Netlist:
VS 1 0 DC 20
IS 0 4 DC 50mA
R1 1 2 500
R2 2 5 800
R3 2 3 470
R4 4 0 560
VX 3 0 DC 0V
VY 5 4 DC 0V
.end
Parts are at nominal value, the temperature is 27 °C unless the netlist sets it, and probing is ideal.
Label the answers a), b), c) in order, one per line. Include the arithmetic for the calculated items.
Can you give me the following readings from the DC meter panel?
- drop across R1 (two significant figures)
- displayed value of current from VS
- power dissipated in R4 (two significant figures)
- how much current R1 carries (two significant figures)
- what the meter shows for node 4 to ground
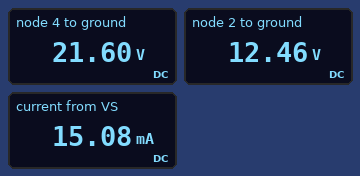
a) 20 V - 12.46 V = 7.5 V
b) 15.08 mA
c) (21.6 V)^2 / 560 Ω = 830 mW
d) (20 V - 12.46 V) / 500 Ω = 15 mA
e) 21.60 V
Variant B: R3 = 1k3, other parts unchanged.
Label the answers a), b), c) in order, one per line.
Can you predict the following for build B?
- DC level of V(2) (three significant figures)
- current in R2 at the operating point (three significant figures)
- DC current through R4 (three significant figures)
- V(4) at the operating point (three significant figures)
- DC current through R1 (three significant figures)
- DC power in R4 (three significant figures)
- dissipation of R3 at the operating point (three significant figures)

a) 17.3 V
b) 7.88 mA
c) 42.1 mA
d) 23.6 V
e) 5.42 mA
f) 994 mW
g) 230 mW
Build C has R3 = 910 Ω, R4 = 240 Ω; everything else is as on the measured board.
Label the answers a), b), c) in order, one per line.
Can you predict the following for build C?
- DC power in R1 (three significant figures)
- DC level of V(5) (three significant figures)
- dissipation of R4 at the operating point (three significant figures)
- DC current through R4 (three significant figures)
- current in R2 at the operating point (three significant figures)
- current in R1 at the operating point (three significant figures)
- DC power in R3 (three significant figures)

a) 107 mW
b) 12.2 V
c) 616 mW
d) 50.7 mA
e) 666 µA
f) 14.6 mA
g) 177 mW
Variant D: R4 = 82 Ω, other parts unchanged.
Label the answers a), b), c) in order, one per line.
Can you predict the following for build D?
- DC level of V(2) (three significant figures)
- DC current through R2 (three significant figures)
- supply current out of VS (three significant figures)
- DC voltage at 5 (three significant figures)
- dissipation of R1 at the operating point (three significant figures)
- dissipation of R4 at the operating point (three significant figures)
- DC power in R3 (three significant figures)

a) 8.49 V
b) 4.97 mA
c) 23.0 mA
d) 4.51 V
e) 265 mW
f) 248 mW
g) 153 mW
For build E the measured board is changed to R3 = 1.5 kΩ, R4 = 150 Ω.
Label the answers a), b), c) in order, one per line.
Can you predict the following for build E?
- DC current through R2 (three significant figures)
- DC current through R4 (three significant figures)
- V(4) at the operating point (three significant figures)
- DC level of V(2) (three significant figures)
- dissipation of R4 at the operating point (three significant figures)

a) 5.66 mA
b) 55.7 mA
c) 8.35 V
d) 12.9 V
e) 465 mW
